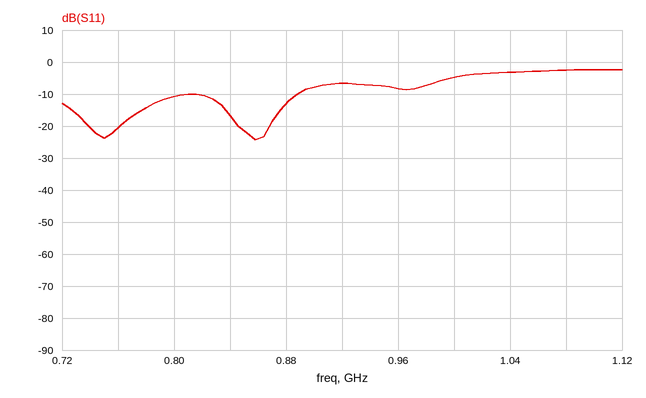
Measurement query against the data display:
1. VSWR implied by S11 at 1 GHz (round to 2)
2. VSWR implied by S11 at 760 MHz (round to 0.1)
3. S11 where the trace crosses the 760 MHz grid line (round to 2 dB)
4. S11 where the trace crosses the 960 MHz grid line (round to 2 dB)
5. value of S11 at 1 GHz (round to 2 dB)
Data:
4
1.2
-20 dB
-8 dB
-4 dB
